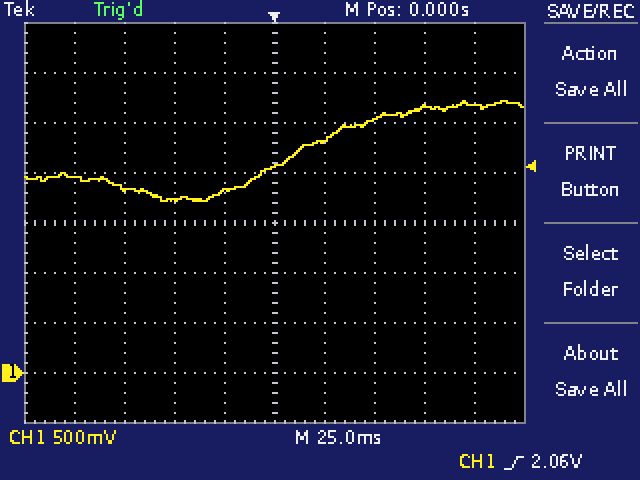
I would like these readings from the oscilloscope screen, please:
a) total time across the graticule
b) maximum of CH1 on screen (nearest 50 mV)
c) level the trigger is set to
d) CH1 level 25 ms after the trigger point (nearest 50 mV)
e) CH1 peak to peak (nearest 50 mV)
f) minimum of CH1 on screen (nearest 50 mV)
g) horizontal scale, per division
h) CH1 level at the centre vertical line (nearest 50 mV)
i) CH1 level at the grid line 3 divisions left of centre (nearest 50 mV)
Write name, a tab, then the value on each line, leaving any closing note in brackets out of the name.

total time across the graticule	250 ms
maximum of CH1 on screen	2.70 V
level the trigger is set to	2.06 V
CH1 level 25 ms after the trigger point	2.35 V
CH1 peak to peak	1.00 V
minimum of CH1 on screen	1.70 V
horizontal scale, per division	25 ms
CH1 level at the centre vertical line	2.05 V
CH1 level at the grid line 3 divisions left of centre	1.85 V
